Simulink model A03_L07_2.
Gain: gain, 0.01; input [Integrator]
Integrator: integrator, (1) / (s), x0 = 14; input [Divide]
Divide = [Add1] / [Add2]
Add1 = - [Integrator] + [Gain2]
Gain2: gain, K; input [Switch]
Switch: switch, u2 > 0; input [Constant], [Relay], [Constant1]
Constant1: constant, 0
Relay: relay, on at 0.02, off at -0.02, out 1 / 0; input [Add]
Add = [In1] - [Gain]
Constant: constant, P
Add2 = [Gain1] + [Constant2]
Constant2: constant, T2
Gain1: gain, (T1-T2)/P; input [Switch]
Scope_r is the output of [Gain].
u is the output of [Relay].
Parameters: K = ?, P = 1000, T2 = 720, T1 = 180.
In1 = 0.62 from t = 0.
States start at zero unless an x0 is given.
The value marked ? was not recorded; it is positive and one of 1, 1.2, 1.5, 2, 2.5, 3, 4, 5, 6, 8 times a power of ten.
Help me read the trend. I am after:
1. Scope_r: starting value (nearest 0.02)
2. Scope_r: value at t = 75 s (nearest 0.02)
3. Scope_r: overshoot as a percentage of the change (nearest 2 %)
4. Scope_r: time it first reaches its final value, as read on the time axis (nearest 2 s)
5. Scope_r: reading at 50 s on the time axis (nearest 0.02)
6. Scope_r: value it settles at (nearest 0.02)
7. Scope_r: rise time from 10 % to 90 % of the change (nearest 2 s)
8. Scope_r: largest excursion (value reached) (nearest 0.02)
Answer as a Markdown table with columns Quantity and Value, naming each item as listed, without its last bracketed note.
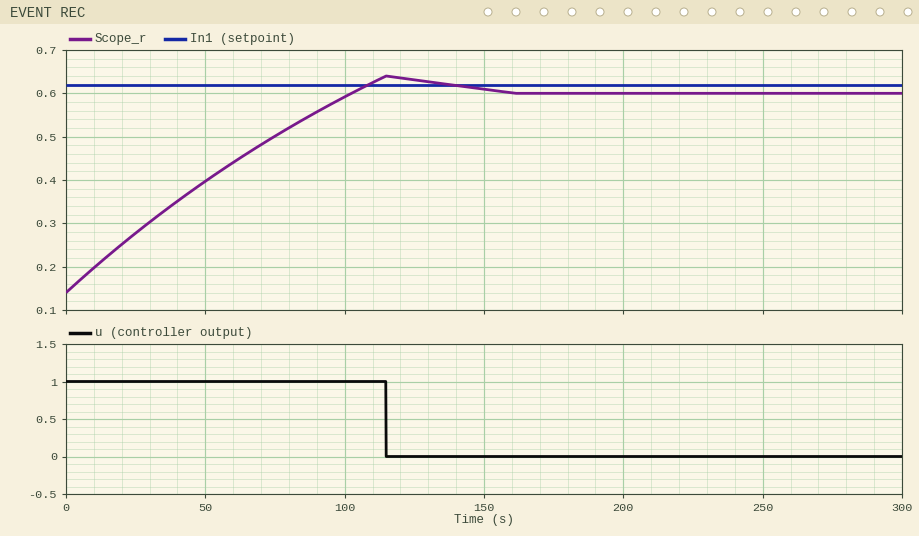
| Quantity | Value |
|---|---|
| Scope_r: starting value | 0.14 |
| Scope_r: value at t = 75 s | 0.50 |
| Scope_r: overshoot as a percentage of the change | 8 % |
| Scope_r: time it first reaches its final value, as read on the time axis | 102 s |
| Scope_r: reading at 50 s on the time axis | 0.40 |
| Scope_r: value it settles at | 0.60 |
| Scope_r: rise time from 10 % to 90 % of the change | 82 s |
| Scope_r: largest excursion (value reached) | 0.64 |
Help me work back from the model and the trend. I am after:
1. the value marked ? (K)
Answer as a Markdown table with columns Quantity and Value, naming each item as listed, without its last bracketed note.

| Quantity | Value |
|---|---|
| the value marked ? | 0.12 |
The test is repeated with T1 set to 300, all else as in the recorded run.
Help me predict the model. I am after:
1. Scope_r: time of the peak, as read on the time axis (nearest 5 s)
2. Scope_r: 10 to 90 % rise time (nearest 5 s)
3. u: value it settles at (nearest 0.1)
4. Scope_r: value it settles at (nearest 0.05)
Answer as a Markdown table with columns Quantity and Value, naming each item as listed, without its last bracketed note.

| Quantity | Value |
|---|---|
| Scope_r: time of the peak, as read on the time axis | 190 s |
| Scope_r: 10 to 90 % rise time | 135 s |
| u: value it settles at | 0.0 |
| Scope_r: value it settles at | 0.60 |
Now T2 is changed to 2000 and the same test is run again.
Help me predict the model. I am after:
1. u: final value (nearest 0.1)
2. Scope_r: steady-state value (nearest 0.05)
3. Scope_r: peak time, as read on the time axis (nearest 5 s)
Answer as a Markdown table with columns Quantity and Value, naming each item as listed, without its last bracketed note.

| Quantity | Value |
|---|---|
| u: final value | 0.0 |
| Scope_r: steady-state value | 0.60 |
| Scope_r: peak time, as read on the time axis | 115 s |
